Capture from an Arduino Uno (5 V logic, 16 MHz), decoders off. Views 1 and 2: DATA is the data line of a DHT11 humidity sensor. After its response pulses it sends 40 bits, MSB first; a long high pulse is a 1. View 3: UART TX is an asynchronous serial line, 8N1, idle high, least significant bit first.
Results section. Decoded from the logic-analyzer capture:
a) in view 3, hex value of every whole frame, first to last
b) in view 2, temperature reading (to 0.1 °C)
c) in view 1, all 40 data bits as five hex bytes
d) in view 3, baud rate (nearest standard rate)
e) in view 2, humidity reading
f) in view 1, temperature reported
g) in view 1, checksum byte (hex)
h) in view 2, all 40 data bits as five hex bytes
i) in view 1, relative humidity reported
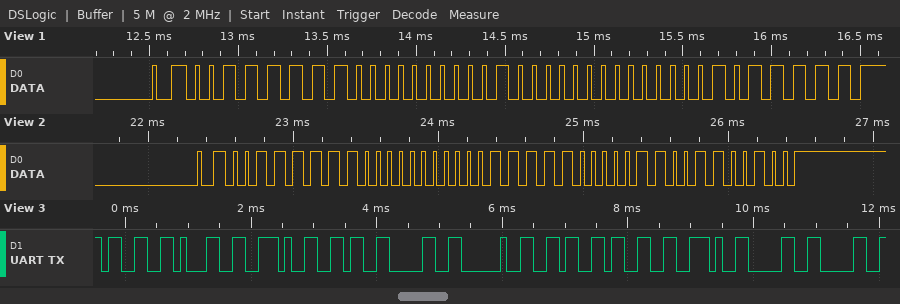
33 31 2E 36 30 20 36 33 2E 30 30
31.6 °C
3F 00 20 00 5F
9600 baud
63 %
32.0 °C
0x5F
3F 00 1F 06 64
63 %
